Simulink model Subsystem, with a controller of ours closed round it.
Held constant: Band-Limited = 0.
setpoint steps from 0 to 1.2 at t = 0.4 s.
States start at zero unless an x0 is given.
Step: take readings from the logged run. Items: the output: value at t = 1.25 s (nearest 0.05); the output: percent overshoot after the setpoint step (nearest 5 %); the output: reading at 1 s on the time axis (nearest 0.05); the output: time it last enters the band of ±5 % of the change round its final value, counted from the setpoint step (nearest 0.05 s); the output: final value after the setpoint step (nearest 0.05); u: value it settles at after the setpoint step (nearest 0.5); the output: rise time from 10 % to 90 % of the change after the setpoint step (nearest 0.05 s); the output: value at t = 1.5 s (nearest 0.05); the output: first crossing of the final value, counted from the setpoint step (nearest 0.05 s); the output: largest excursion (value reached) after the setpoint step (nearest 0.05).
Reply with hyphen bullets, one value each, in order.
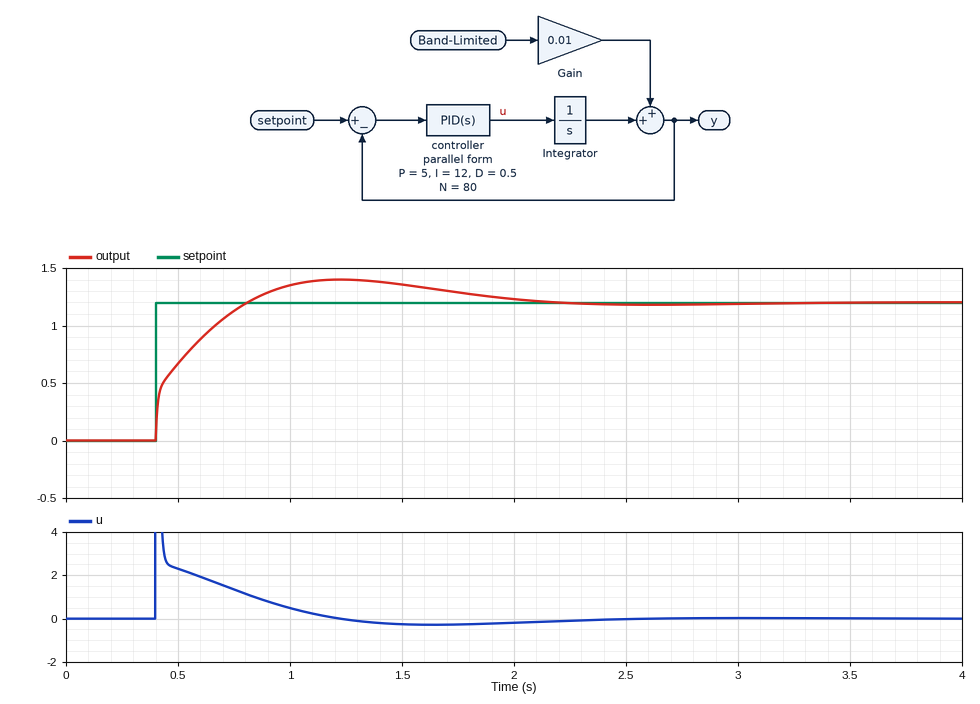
- 1.40
- 15 %
- 1.35
- 1.45 s
- 1.20
- 0.0
- 0.30 s
- 1.35
- 0.40 s
- 1.40
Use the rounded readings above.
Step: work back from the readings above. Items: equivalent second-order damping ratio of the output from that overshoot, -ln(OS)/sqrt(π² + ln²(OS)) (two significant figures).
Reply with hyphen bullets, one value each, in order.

- 0.52
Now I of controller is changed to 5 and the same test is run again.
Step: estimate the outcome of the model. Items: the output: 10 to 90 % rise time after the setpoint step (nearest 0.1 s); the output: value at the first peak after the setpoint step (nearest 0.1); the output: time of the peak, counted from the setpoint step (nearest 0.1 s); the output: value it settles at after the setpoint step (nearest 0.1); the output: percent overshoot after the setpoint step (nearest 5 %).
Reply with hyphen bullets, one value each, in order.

- 0.4 s
- 1.3
- 1.1 s
- 1.2
- 10 %
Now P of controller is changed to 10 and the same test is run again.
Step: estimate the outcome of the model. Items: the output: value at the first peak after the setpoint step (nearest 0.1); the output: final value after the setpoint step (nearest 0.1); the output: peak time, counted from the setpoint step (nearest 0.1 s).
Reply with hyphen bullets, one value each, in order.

- 1.3
- 1.2
- 0.7 s
